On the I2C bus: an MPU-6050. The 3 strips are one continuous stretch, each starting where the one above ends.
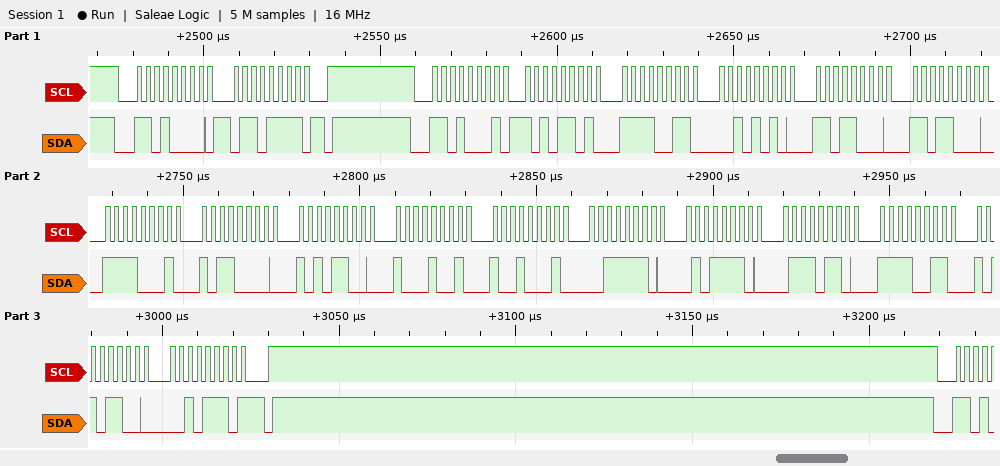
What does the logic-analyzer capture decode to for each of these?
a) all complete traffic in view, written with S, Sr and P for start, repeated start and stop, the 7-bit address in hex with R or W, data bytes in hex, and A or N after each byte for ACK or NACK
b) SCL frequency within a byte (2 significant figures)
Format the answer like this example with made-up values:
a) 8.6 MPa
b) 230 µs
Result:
a) S 68W A 6F A P S 68R A AD A F3 A 2A A D8 A D8 A F1 A B0 A AC A 89 A 91 A 3E A 5E A 76 A F3 A AC A 2E N P
b) 400 kHz
